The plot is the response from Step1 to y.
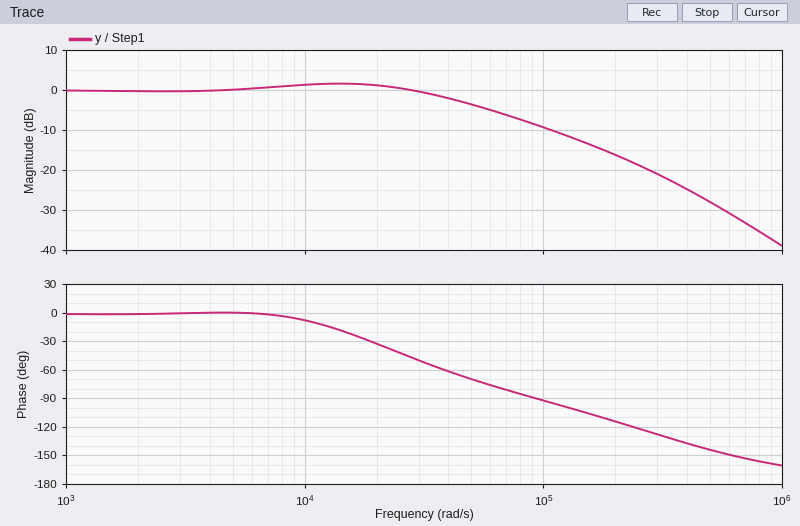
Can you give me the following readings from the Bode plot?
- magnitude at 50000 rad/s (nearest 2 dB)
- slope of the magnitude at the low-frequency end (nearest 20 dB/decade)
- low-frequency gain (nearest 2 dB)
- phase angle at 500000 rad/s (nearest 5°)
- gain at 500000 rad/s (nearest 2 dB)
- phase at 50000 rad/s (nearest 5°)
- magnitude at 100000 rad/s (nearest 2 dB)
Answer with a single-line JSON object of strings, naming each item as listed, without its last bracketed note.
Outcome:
{"magnitude at 50000 rad/s": "-4 dB", "slope of the magnitude at the low-frequency end": "0 dB/decade", "low-frequency gain": "0 dB", "phase angle at 500000 rad/s": "-145°", "gain at 500000 rad/s": "-28 dB", "phase at 50000 rad/s": "-70°", "magnitude at 100000 rad/s": "-10 dB"}
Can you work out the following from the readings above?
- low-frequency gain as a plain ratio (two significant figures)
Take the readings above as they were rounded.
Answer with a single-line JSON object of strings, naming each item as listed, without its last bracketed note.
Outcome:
{"low-frequency gain as a plain ratio": "1.0"}
